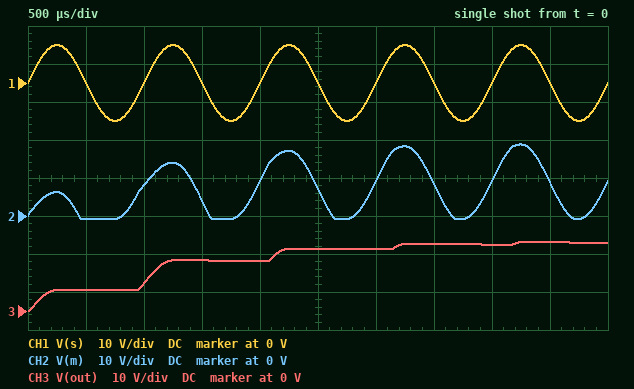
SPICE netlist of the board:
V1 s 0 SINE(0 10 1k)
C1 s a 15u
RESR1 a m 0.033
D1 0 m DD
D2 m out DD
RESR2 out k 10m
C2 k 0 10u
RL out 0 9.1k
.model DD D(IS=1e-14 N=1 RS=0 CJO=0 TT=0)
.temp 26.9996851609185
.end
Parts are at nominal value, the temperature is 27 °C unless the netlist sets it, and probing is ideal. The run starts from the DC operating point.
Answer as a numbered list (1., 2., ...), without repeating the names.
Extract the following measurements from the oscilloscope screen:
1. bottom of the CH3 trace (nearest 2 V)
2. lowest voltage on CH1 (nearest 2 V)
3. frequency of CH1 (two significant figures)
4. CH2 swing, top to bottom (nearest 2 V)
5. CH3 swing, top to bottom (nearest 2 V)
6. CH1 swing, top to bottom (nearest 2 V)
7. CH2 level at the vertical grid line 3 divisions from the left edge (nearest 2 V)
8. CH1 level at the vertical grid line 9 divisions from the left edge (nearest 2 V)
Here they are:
1. 0 V
2. -10 V
3. 1.0 kHz
4. 20 V
5. 18 V
6. 20 V
7. 4 V
8. 0 V
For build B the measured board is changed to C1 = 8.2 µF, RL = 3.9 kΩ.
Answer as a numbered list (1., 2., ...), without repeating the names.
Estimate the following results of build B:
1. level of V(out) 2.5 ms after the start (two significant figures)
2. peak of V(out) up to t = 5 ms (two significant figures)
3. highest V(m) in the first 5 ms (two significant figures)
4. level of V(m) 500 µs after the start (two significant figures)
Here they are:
1. 14 V
2. 17 V
3. 18 V
4. -820 mV
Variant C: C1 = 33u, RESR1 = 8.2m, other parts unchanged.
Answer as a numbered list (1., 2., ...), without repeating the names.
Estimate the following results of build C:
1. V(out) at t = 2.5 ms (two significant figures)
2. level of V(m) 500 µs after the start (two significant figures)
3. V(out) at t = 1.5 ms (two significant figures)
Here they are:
1. 18 V
2. -850 mV
3. 16 V
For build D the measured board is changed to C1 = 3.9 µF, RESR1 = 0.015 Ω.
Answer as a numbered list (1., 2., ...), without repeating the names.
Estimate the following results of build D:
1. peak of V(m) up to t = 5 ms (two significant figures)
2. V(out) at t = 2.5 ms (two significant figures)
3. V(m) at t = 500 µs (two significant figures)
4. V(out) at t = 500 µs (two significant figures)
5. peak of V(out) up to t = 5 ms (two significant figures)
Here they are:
1. 15 V
2. 10 V
3. -800 mV
4. 2.6 V
5. 14 V
